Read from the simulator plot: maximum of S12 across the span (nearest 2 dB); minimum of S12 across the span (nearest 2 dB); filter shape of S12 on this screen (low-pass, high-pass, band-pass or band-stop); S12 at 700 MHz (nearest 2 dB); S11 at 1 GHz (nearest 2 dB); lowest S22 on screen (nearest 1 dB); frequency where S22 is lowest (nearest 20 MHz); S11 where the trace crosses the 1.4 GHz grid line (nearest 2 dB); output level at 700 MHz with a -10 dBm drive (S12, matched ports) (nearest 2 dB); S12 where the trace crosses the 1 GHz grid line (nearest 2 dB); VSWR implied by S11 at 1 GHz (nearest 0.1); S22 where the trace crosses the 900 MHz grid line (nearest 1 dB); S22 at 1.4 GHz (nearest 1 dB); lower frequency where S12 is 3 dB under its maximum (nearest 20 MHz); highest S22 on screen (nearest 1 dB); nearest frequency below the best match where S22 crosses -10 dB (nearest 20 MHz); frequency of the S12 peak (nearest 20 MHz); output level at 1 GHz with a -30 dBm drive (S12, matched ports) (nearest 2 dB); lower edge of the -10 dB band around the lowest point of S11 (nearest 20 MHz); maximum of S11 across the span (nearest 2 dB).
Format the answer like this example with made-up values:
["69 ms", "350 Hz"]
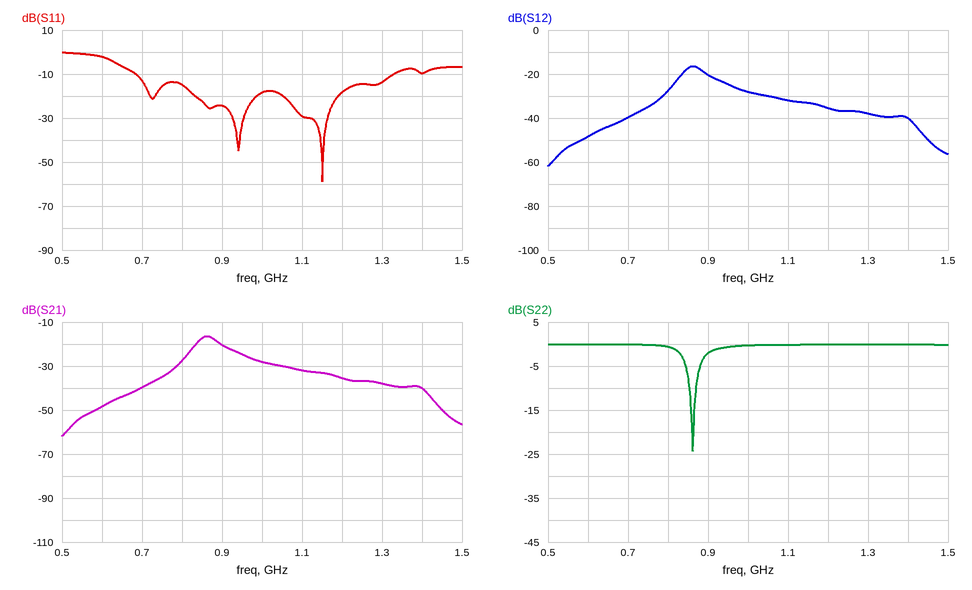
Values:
["-16 dB", "-62 dB", "band-pass", "-40 dB", "-18 dB", "-24 dB", "860 MHz", "-10 dB", "-50 dBm", "-28 dB", "1.3", "-2 dB", "0 dB", "840 MHz", "0 dB", "860 MHz", "860 MHz", "-58 dBm", "680 MHz", "0 dB"]
